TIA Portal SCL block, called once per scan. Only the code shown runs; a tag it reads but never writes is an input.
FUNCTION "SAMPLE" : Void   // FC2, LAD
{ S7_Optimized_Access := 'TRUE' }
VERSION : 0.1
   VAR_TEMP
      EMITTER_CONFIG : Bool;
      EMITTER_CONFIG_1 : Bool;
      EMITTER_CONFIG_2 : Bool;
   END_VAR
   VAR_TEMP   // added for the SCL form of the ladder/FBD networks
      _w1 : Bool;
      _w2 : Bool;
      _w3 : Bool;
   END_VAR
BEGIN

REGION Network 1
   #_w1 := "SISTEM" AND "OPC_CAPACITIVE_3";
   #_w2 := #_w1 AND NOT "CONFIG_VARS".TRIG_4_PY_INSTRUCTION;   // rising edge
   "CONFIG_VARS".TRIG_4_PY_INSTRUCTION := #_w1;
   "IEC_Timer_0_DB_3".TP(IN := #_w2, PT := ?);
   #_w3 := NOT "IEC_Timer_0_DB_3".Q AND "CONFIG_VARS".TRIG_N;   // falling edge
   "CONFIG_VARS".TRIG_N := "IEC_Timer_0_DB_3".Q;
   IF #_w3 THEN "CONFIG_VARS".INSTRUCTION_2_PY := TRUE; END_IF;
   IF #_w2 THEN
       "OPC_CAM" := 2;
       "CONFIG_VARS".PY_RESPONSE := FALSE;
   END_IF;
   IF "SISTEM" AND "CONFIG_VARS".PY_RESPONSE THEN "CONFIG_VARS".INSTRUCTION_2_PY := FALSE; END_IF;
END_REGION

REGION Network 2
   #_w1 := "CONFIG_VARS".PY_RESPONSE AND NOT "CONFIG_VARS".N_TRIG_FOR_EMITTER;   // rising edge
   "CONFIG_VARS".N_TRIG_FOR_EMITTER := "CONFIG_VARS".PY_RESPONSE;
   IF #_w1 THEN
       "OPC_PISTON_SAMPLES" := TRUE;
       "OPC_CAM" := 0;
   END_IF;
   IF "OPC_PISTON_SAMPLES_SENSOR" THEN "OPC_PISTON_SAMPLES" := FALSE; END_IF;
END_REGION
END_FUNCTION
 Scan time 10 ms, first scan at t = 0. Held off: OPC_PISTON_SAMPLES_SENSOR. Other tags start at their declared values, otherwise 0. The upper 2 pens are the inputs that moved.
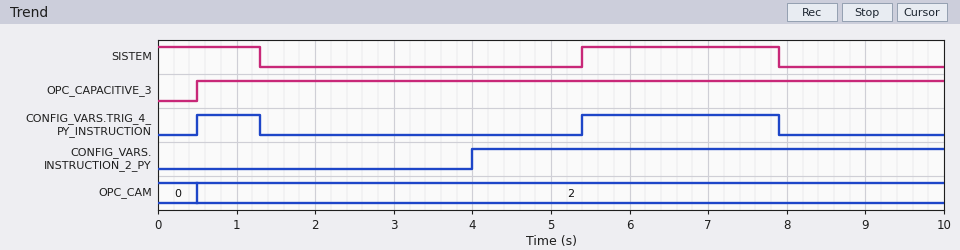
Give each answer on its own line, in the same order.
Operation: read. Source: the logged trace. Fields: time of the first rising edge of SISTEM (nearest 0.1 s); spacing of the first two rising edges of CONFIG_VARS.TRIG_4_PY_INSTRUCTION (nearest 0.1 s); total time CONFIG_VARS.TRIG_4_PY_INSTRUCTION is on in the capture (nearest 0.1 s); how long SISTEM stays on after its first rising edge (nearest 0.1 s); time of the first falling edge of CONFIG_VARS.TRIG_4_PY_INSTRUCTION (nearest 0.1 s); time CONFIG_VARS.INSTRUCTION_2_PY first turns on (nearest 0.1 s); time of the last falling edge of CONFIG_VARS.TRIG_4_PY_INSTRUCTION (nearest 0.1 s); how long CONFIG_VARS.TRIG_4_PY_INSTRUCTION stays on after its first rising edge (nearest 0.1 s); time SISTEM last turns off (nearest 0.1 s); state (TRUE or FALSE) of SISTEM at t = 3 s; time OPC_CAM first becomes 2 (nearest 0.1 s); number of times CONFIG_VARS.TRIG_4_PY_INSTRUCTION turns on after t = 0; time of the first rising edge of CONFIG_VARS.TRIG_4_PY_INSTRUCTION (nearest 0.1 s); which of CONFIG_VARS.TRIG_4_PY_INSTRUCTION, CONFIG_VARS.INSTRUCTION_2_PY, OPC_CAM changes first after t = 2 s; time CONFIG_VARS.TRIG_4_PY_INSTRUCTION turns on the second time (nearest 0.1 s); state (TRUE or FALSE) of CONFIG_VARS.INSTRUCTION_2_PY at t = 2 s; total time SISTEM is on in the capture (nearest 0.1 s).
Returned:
5.4 s
4.9 s
3.3 s
2.5 s
1.3 s
4.0 s
7.9 s
0.8 s
7.9 s
FALSE
0.5 s
2
0.5 s
CONFIG_VARS.INSTRUCTION_2_PY
5.4 s
FALSE
3.8 s
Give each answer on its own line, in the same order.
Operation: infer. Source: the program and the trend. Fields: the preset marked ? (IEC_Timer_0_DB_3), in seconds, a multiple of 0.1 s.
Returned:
3.5 s
